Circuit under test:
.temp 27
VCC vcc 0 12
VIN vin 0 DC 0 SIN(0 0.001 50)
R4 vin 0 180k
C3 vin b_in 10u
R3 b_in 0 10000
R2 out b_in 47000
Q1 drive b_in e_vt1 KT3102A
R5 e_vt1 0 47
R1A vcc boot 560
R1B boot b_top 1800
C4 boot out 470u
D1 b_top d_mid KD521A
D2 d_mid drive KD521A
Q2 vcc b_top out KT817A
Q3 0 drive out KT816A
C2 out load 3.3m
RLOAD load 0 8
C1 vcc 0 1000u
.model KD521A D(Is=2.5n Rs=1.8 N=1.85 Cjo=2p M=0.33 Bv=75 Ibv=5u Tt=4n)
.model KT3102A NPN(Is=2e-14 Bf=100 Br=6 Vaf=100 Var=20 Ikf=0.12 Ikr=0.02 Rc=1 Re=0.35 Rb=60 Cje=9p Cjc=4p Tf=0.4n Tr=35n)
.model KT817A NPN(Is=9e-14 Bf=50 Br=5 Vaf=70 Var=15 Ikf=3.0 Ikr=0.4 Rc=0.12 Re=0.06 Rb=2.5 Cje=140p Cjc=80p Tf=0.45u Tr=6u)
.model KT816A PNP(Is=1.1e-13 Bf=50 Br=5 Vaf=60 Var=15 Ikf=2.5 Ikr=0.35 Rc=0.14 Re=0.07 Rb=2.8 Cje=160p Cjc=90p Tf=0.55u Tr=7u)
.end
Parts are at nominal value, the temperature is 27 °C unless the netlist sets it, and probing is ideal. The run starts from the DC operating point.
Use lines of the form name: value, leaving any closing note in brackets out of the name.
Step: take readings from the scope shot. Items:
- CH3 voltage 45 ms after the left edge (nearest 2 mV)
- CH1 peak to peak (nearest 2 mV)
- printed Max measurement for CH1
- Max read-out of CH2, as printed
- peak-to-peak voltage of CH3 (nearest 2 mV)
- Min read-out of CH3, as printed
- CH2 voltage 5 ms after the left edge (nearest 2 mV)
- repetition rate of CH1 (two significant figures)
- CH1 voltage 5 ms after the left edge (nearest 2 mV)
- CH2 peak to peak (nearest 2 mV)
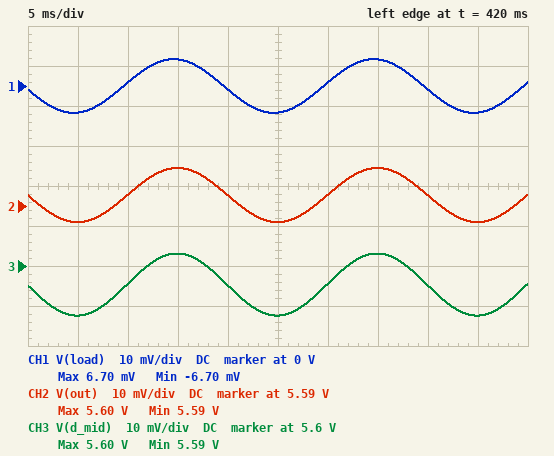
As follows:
CH3 voltage 45 ms after the left edge: 5.588 V
CH1 peak to peak: 14 mV
printed Max measurement for CH1: 6.70 mV
Max read-out of CH2, as printed: 5.60 V
peak-to-peak voltage of CH3: 16 mV
Min read-out of CH3, as printed: 5.59 V
CH2 voltage 5 ms after the left edge: 5.586 V
repetition rate of CH1: 50 Hz
CH1 voltage 5 ms after the left edge: -6 mV
CH2 peak to peak: 14 mV
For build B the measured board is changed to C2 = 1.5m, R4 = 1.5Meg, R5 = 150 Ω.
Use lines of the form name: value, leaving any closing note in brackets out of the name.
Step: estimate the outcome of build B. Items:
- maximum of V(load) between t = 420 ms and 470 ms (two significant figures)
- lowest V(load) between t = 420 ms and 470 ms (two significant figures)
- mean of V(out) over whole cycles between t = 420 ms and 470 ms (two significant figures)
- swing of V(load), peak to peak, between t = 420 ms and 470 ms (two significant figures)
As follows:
maximum of V(load) between t = 420 ms and 470 ms: 2.4 mV
lowest V(load) between t = 420 ms and 470 ms: -2.4 mV
mean of V(out) over whole cycles between t = 420 ms and 470 ms: 6.5 V
swing of V(load), peak to peak, between t = 420 ms and 470 ms: 4.8 mV
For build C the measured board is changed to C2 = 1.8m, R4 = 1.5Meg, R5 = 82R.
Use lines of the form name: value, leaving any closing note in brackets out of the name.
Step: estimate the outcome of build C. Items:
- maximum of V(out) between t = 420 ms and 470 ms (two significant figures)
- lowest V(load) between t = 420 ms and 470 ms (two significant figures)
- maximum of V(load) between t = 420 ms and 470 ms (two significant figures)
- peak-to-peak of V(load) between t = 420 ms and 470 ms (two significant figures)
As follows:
maximum of V(out) between t = 420 ms and 470 ms: 5.9 V
lowest V(load) between t = 420 ms and 470 ms: -4.2 mV
maximum of V(load) between t = 420 ms and 470 ms: 4.2 mV
peak-to-peak of V(load) between t = 420 ms and 470 ms: 8.4 mV
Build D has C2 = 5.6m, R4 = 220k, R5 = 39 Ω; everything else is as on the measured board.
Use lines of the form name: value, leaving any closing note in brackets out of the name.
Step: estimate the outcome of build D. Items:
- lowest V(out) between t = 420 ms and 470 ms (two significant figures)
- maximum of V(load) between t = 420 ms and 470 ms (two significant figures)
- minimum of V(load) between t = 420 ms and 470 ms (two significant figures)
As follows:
lowest V(out) between t = 420 ms and 470 ms: 5.5 V
maximum of V(load) between t = 420 ms and 470 ms: 7.8 mV
minimum of V(load) between t = 420 ms and 470 ms: -7.8 mV
